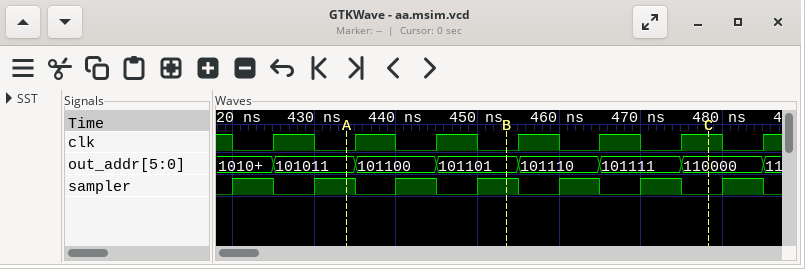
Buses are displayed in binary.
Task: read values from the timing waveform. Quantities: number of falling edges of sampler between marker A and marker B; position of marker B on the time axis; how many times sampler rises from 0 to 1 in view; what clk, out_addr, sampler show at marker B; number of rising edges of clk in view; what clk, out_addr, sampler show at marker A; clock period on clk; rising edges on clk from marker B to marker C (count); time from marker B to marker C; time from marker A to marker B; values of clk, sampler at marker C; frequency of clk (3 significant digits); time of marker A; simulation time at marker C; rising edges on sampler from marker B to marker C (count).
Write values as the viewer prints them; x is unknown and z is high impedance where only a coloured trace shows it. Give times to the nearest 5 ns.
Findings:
2
455 ns
7
clk=0, out_addr=101101, sampler=1
7
clk=0, out_addr=101011, sampler=1
10 ns
3
25 ns
20 ns
clk=1, sampler=0
100 MHz
435 ns
480 ns
2
